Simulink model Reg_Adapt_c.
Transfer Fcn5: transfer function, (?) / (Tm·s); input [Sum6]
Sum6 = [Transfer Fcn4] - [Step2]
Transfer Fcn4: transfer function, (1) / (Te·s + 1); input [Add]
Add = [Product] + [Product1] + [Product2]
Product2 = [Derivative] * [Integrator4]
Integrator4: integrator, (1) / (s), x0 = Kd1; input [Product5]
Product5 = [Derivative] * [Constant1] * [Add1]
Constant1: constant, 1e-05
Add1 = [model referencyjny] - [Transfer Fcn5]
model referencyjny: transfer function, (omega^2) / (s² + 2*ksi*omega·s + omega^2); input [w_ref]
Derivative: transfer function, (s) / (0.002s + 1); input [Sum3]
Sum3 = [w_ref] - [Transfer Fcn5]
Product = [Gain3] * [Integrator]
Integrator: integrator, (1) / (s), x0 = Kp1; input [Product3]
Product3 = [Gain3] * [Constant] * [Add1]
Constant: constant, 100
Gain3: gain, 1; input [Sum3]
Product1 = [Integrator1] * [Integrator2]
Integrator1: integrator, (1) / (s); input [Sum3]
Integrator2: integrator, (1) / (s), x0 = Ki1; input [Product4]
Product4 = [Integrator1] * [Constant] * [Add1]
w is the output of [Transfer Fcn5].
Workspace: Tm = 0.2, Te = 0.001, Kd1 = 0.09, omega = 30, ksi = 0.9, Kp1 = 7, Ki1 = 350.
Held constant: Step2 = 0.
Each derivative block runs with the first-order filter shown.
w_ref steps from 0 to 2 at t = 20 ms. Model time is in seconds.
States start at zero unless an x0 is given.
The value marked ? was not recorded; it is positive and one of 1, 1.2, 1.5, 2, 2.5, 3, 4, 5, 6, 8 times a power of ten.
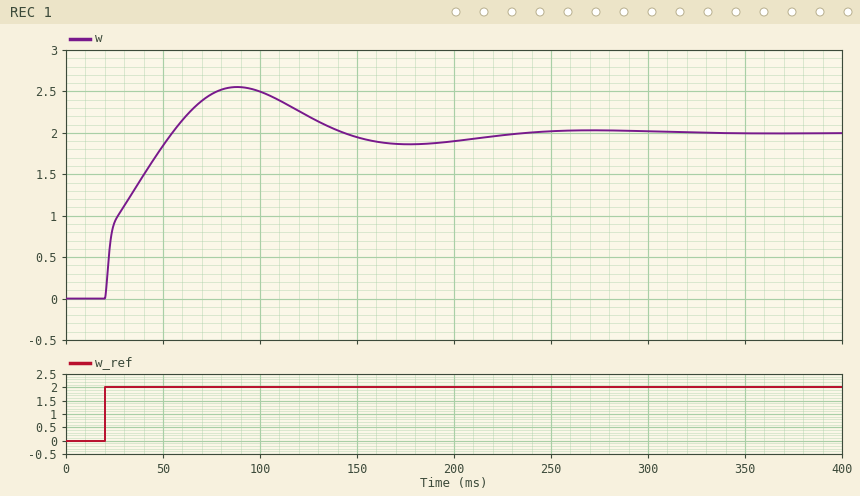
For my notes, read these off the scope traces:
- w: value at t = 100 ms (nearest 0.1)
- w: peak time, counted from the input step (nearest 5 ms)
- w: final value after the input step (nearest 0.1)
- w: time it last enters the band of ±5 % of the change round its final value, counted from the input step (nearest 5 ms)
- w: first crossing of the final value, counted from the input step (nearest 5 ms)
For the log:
2.5
70 ms
2.0
180 ms
35 ms
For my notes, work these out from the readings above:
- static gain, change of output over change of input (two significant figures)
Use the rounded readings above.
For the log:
1.0
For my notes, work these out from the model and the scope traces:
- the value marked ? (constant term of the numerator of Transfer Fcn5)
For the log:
1.2
